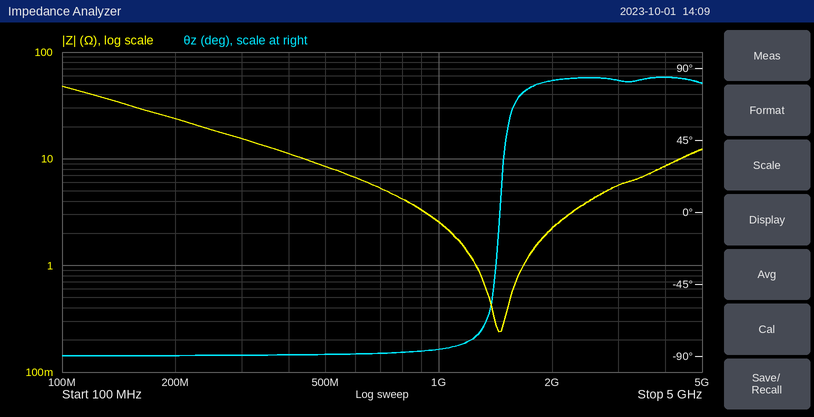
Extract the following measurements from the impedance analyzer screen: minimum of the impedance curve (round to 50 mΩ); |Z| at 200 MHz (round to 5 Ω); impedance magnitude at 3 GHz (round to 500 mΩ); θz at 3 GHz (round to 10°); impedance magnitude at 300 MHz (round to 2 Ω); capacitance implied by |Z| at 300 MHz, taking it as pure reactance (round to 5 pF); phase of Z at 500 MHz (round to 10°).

250 mΩ
25 Ω
5.5 Ω
80°
16 Ω
35 pF
-90°
